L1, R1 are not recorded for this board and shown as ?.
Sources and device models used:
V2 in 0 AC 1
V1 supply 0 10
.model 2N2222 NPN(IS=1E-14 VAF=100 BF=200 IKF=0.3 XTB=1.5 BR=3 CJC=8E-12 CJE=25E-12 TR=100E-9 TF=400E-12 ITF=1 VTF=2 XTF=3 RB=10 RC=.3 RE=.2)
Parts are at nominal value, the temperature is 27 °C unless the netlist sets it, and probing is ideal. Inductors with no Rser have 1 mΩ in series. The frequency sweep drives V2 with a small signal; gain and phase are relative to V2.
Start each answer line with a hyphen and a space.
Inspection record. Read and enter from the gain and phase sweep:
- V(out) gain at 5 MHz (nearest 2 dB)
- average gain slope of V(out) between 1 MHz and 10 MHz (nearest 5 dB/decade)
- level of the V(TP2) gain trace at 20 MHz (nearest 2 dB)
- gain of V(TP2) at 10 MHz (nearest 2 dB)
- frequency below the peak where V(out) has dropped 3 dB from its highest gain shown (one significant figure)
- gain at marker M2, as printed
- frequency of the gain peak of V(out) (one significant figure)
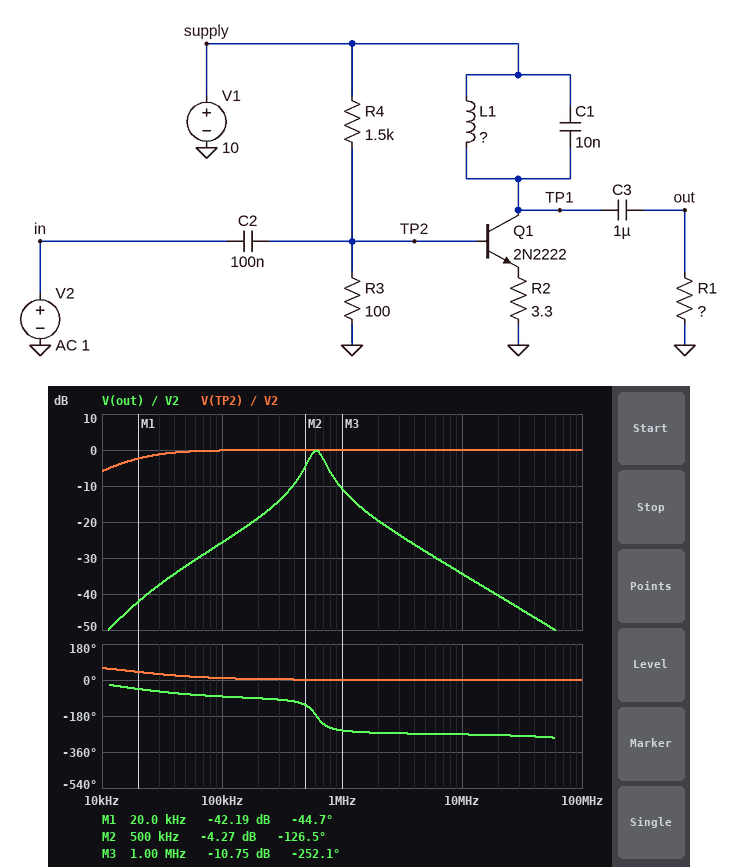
- -28 dB
- -25 dB/decade
- 0 dB
- 0 dB
- 500 kHz
- -4.27 dB
- 600 kHz
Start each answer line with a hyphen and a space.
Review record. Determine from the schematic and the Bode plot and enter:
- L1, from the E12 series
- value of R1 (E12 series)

- 6.8 µH
- 82 Ω
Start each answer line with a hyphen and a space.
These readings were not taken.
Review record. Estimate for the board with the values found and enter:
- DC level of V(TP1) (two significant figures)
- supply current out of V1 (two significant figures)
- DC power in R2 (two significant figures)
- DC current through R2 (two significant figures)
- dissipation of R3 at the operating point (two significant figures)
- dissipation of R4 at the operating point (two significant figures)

- 10 V
- 6.6 mA
- 350 nW
- 330 µA
- 3.9 mW
- 59 mW
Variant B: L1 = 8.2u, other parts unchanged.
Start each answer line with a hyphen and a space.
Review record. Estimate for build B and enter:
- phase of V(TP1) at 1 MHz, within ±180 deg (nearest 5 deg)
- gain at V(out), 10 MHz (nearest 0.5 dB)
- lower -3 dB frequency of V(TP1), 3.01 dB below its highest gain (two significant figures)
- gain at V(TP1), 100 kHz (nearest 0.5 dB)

- 105 deg
- -34.5 dB
- 470 kHz
- -24.0 dB
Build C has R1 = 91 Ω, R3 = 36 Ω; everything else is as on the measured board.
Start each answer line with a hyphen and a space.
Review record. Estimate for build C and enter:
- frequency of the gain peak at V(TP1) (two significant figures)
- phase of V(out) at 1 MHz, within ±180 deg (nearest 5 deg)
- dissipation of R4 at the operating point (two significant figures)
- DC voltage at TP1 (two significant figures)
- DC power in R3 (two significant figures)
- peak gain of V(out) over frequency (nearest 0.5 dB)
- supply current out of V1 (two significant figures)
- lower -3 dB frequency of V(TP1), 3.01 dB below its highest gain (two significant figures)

- 620 kHz
- 20 deg
- 64 mW
- 10 V
- 1.5 mW
- -58.5 dB
- 6.5 mA
- 550 kHz
